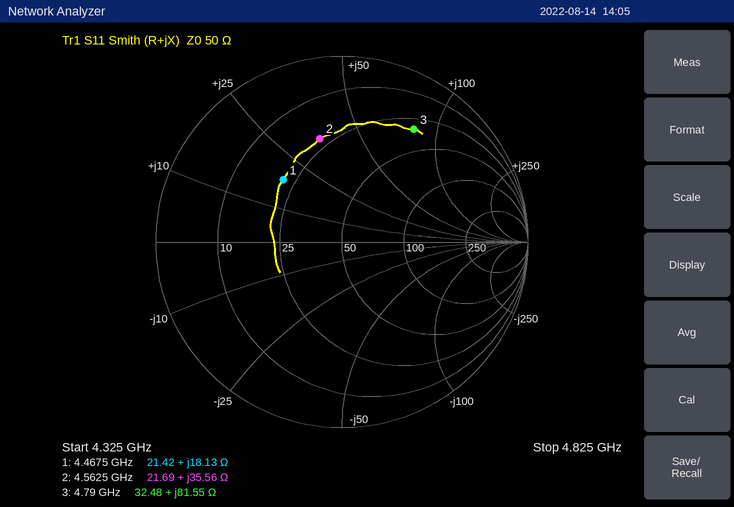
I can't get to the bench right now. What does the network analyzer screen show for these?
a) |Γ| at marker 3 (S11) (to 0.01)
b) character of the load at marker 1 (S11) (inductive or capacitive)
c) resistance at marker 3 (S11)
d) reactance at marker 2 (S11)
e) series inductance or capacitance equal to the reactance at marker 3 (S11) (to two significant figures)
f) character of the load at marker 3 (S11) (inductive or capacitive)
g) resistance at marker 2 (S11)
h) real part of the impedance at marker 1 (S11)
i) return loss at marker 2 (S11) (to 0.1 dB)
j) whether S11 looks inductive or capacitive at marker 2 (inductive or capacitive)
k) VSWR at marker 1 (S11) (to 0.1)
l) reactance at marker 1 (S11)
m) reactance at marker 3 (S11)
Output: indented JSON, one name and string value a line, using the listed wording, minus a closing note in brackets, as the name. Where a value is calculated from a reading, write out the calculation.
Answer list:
{
  "|Γ| at marker 3 (S11)": "0.72",
  "character of the load at marker 1 (S11)": "inductive",
  "resistance at marker 3": "32.48 Ω",
  "reactance at marker 2": "+35.56 Ω",
  "series inductance or capacitance equal to the reactance at marker 3 (S11)": "L = 81.55 Ω/(2π × 4.79 GHz) ≈ 2.7 nH",
  "character of the load at marker 3 (S11)": "inductive",
  "resistance at marker 2": "21.69 Ω",
  "real part of the impedance at marker 1": "21.42 Ω",
  "return loss at marker 2 (S11)": "4.9 dB",
  "whether S11 looks inductive or capacitive at marker 2": "inductive",
  "VSWR at marker 1 (S11)": "2.7",
  "reactance at marker 1": "+18.13 Ω",
  "reactance at marker 3": "+81.55 Ω"
}
